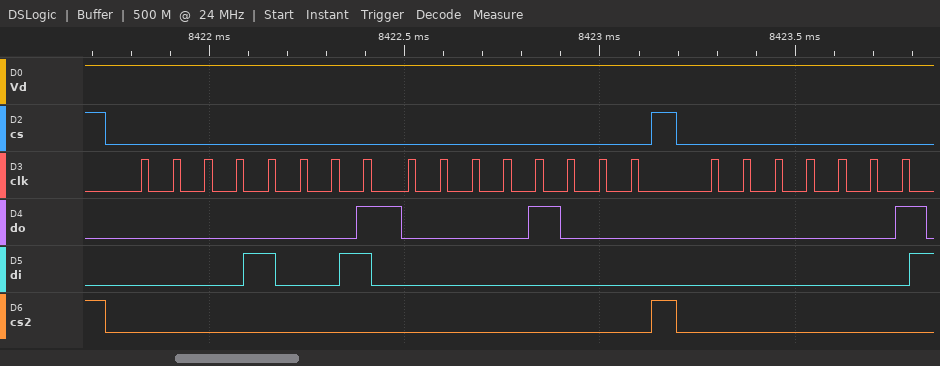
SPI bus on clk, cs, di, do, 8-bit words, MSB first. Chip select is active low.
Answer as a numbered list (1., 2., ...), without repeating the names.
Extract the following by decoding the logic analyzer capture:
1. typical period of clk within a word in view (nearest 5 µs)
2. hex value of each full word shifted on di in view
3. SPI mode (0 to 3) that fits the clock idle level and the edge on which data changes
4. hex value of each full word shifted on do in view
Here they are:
1. 80 µs
2. 09, 00
3. 0
4. 01, 08
